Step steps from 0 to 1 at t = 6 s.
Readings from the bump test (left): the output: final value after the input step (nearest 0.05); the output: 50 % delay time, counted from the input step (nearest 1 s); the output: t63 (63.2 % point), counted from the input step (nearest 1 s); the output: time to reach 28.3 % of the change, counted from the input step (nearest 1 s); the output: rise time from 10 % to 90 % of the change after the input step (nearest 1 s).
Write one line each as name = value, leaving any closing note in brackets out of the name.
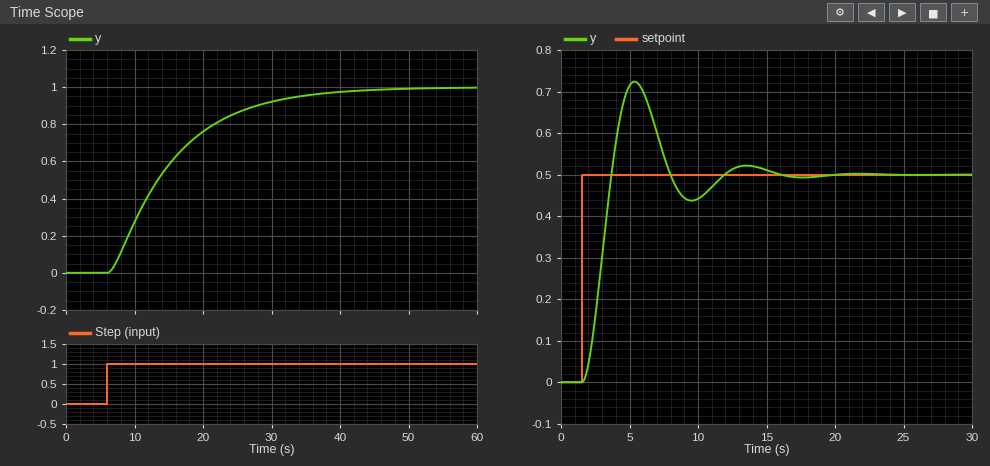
the output: final value after the input step = 1.00
the output: 50 % delay time, counted from the input step = 7 s
the output: t63 (63.2 % point), counted from the input step = 10 s
the output: time to reach 28.3 % of the change, counted from the input step = 4 s
the output: rise time from 10 % to 90 % of the change after the input step = 20 s
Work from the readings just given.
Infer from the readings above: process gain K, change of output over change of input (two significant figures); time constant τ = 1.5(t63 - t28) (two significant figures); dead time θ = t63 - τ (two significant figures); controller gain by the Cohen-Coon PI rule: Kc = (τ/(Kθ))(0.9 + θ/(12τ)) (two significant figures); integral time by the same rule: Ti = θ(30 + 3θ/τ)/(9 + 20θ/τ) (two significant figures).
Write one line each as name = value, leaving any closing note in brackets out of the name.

process gain K, change of output over change of input = 1.0
time constant τ = 1.5(t63 - t28) = 9.0 s
dead time θ = t63 - τ = 1.0 s
controller gain by the Cohen-Coon PI rule: Kc = (τ/(Kθ))(0.9 + θ/(12τ)) = 8.2
integral time by the same rule: Ti = θ(30 + 3θ/τ)/(9 + 20θ/τ) = 2.7 s
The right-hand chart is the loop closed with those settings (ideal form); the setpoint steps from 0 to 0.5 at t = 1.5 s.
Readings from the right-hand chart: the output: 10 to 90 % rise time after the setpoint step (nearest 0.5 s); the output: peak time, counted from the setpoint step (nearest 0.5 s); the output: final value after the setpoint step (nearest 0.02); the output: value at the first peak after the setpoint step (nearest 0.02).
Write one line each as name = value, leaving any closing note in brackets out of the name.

the output: 10 to 90 % rise time after the setpoint step = 1.5 s
the output: peak time, counted from the setpoint step = 4.0 s
the output: final value after the setpoint step = 0.50
the output: value at the first peak after the setpoint step = 0.72
